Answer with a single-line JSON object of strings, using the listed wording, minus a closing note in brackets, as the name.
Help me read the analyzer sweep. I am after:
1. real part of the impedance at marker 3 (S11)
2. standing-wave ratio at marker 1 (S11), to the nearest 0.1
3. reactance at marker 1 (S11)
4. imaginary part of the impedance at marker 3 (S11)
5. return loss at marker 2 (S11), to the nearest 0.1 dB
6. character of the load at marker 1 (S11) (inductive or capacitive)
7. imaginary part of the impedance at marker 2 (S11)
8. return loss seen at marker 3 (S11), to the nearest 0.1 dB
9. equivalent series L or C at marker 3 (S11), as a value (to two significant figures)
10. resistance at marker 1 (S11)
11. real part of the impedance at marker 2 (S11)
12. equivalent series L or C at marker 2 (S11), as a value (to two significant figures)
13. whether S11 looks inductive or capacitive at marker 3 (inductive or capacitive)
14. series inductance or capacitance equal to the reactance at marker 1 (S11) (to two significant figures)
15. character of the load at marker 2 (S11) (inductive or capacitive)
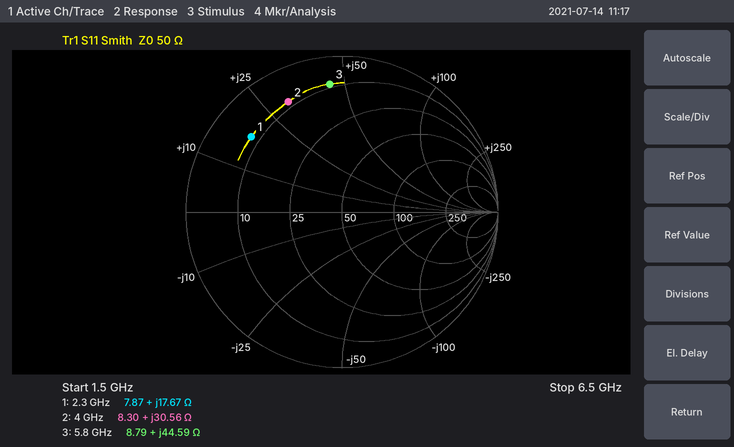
{"real part of the impedance at marker 3": "8.79 Ω", "standing-wave ratio at marker 1 (S11), to the nearest 0.1": "7.2", "reactance at marker 1": "+17.67 Ω", "imaginary part of the impedance at marker 3": "+44.59 Ω", "return loss at marker 2 (S11), to the nearest 0.1 dB": "2.1 dB", "character of the load at marker 1 (S11)": "inductive", "imaginary part of the impedance at marker 2": "+30.56 Ω", "return loss seen at marker 3 (S11), to the nearest 0.1 dB": "1.7 dB", "equivalent series L or C at marker 3 (S11), as a value": "1.2 nH", "resistance at marker 1": "7.87 Ω", "real part of the impedance at marker 2": "8.30 Ω", "equivalent series L or C at marker 2 (S11), as a value": "1.2 nH", "whether S11 looks inductive or capacitive at marker 3": "inductive", "series inductance or capacitance equal to the reactance at marker 1 (S11)": "1.2 nH", "character of the load at marker 2 (S11)": "inductive"}
